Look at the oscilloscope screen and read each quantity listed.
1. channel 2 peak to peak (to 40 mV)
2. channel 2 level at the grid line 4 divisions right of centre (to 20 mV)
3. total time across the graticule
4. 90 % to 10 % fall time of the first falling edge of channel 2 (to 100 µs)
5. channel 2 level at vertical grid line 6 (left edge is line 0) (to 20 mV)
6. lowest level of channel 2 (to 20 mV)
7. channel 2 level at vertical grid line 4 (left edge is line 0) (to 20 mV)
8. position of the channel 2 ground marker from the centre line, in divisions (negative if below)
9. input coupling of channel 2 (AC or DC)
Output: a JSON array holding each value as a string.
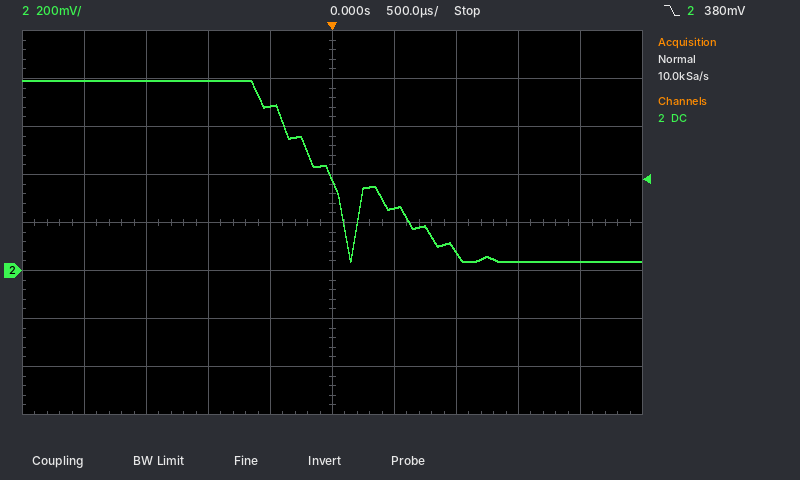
["760 mV", "40 mV", "5 ms", "700 µs", "260 mV", "40 mV", "680 mV", "-1.0 div", "DC"]
